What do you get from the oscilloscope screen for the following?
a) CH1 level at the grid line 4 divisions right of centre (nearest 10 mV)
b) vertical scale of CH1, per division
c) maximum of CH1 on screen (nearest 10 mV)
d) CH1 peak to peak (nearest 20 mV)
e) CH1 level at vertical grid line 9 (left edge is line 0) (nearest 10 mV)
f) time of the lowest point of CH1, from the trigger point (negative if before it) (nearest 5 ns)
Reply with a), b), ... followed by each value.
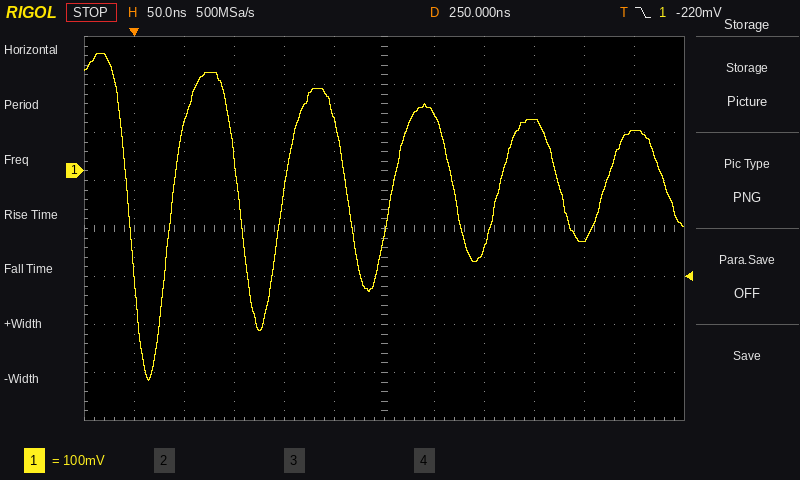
a) -140 mV
b) 100 mV
c) 240 mV
d) 680 mV
e) 110 mV
f) +15 ns
